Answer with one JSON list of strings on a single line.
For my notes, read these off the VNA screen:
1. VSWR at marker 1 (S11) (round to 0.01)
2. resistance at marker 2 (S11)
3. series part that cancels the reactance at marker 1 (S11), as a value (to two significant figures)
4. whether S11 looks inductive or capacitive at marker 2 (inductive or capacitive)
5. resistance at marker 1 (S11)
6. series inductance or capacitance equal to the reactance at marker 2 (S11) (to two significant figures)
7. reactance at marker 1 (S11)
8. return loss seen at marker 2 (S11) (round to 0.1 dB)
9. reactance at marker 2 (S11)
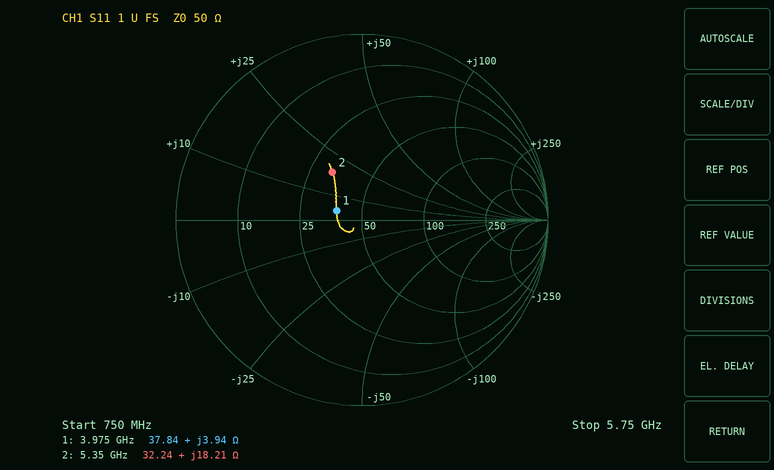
["1.34", "32.24 Ω", "10 pF", "inductive", "37.84 Ω", "540 pH", "+3.94 Ω", "10.4 dB", "+18.21 Ω"]
